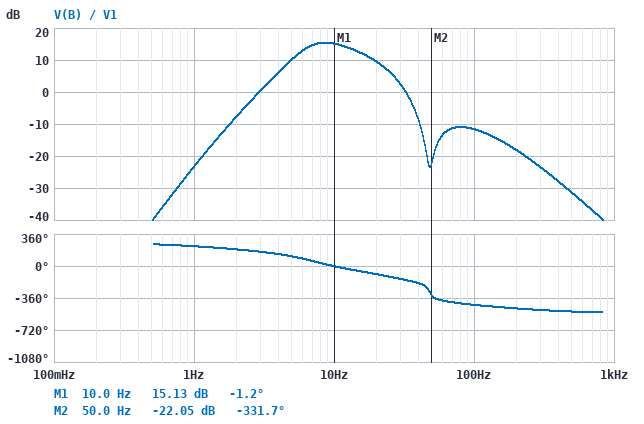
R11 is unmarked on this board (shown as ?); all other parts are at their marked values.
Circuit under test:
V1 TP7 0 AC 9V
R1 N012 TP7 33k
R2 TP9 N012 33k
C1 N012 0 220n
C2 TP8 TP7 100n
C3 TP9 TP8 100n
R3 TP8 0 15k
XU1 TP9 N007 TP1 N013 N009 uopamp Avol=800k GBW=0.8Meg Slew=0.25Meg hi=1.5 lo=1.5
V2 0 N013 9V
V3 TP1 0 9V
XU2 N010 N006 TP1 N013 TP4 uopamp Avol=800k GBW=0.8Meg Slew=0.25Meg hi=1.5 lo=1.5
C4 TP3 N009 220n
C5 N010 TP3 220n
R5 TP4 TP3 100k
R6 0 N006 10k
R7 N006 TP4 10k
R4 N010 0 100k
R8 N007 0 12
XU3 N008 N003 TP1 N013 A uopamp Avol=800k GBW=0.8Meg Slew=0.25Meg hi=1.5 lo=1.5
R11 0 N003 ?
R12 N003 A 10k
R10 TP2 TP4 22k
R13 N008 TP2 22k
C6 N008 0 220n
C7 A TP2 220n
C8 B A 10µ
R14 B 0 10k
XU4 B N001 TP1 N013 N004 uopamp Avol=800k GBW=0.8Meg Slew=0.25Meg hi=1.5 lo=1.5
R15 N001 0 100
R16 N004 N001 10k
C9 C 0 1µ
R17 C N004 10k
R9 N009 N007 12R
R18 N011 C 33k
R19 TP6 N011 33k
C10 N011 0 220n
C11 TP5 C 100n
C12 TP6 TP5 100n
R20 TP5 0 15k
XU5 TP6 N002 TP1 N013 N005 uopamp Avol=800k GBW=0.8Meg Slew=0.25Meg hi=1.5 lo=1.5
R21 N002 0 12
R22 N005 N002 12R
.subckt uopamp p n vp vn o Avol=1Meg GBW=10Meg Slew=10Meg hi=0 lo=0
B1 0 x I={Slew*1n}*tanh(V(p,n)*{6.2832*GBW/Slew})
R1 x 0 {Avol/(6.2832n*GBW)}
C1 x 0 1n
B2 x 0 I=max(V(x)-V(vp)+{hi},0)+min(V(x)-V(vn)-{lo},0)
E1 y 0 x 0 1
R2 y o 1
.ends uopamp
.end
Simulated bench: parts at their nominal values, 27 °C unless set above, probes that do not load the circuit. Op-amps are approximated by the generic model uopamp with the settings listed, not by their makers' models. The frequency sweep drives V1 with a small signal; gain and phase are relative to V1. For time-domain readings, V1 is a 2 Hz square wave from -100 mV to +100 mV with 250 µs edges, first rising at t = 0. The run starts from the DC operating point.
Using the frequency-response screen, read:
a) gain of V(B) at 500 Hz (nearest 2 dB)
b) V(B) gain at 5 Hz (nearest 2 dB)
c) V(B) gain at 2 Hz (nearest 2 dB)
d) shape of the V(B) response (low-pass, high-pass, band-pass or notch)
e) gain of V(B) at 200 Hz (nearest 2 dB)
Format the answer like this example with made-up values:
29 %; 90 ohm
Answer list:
-32 dB; 10 dB; -8 dB; band-pass; -18 dB
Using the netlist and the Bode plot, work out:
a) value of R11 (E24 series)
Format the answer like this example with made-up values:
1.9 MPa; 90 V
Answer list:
15 kΩ
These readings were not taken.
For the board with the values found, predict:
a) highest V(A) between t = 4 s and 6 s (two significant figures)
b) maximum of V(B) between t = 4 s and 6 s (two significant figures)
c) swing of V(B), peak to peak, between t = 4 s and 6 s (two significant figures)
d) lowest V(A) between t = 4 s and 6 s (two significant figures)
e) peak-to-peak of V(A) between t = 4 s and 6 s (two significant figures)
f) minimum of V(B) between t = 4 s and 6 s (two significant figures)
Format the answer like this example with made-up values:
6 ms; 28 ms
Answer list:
520 mV; 450 mV; 910 mV; -520 mV; 1.0 V; -450 mV
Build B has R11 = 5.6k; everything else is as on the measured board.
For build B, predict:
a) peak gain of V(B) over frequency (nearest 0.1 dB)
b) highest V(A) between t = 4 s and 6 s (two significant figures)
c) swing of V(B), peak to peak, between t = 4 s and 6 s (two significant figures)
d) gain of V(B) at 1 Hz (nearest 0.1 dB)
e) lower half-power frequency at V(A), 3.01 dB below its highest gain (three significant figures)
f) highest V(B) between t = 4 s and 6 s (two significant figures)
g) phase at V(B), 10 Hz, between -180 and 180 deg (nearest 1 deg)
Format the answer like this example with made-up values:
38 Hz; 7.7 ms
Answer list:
20.7 dB; 1.2 V; 2.1 V; -18.9 dB; 5.88 Hz; 1.1 V; 19 deg
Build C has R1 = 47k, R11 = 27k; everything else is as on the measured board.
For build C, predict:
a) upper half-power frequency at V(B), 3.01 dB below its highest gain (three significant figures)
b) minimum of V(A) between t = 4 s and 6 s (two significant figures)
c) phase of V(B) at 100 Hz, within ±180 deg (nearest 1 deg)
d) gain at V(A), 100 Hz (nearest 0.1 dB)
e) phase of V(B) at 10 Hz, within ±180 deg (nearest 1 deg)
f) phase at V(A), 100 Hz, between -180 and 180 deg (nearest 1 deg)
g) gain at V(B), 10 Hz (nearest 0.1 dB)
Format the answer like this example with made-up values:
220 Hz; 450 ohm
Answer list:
13.4 Hz; -350 mV; -72 deg; -13.1 dB; -15 deg; -73 deg; 11.8 dB
